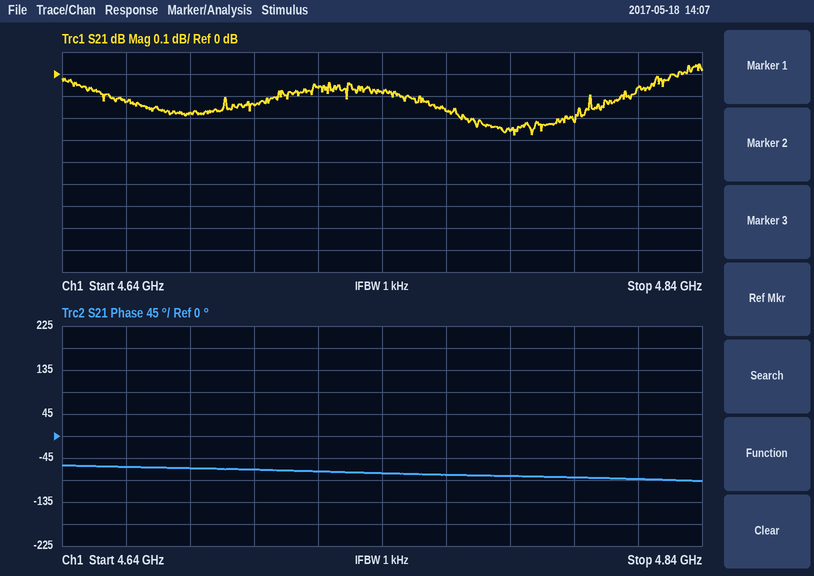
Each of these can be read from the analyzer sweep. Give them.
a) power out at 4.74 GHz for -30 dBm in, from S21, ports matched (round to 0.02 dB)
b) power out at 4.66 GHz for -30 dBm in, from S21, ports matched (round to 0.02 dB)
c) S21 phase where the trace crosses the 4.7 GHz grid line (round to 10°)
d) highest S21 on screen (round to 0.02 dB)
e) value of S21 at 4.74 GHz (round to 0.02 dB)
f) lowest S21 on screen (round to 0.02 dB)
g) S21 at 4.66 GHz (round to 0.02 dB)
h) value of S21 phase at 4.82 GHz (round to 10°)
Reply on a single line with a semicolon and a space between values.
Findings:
-30.08 dBm; -30.12 dBm; -70°; 0.04 dB; -0.08 dB; -0.28 dB; -0.12 dB; -90°
